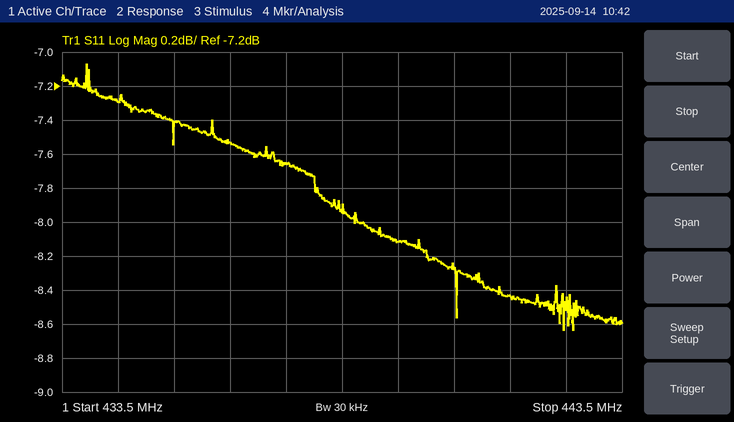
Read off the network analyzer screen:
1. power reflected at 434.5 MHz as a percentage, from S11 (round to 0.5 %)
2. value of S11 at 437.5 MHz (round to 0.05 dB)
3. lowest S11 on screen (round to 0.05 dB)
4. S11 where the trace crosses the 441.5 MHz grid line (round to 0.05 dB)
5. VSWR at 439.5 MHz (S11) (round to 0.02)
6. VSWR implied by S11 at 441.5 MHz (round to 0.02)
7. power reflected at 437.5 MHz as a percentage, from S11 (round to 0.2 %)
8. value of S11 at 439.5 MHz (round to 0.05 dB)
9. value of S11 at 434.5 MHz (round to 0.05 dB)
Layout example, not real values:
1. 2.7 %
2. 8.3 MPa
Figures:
1. 18.5 %
2. -7.65 dB
3. -8.65 dB
4. -8.45 dB
5. 2.30
6. 2.22
7. 17.2 %
8. -8.10 dB
9. -7.30 dB
